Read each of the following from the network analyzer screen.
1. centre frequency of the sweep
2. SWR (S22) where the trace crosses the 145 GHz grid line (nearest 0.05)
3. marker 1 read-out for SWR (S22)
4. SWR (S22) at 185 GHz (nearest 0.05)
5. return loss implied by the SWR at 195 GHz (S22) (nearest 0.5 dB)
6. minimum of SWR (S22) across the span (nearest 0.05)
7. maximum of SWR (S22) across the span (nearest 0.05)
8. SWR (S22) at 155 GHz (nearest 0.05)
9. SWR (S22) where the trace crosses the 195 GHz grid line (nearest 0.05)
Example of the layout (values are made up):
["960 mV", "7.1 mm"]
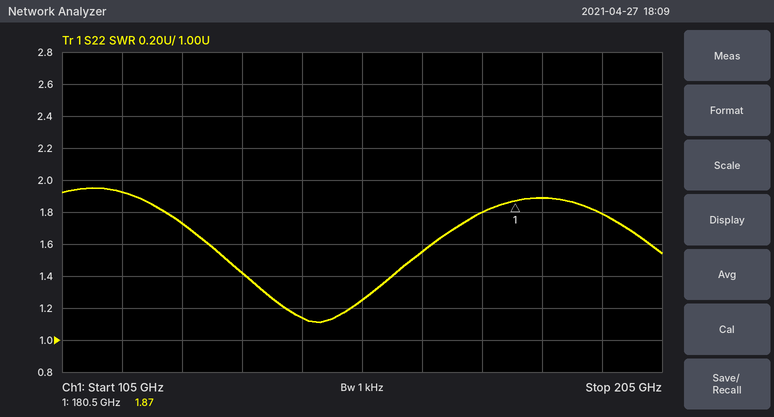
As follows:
["155 GHz", "1.15", "1.87", "1.90", "11.0 dB", "1.10", "1.95", "1.25", "1.80"]
